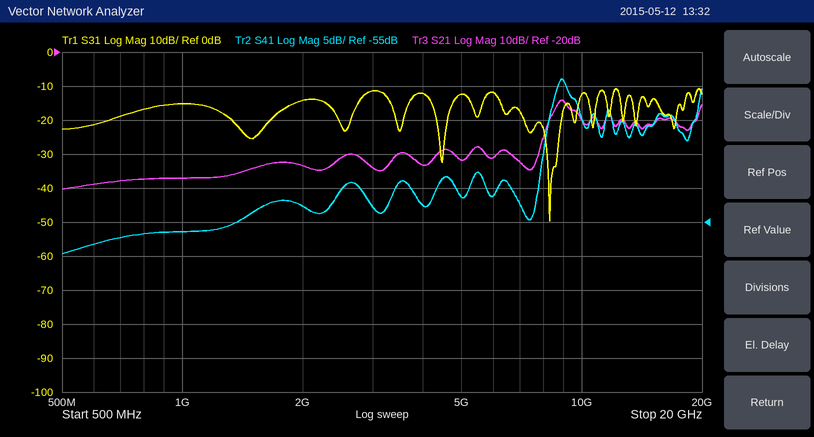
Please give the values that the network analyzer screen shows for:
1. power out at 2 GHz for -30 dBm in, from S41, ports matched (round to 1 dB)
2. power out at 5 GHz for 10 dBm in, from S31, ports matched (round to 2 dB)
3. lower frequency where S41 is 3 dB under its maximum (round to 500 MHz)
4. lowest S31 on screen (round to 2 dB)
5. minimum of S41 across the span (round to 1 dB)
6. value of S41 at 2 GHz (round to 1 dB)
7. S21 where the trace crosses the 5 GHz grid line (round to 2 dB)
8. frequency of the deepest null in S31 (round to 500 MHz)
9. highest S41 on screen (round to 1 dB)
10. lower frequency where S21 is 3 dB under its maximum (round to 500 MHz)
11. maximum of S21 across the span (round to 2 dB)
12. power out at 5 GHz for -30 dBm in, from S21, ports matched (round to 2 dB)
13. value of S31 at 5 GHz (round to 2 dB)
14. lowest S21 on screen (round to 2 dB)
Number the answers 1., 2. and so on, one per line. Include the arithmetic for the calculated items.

1. -30 dBm + (-53 dB) = -83 dBm
2. 10 dBm + (-12 dB) = -2 dBm
3. 8.5 GHz
4. -50 dB
5. -60 dB
6. -53 dB
7. -52 dB
8. 8.5 GHz
9. -34 dB
10. 8.5 GHz
11. -34 dB
12. -30 dBm + (-52 dB) = -82 dBm
13. -12 dB
14. -60 dB
